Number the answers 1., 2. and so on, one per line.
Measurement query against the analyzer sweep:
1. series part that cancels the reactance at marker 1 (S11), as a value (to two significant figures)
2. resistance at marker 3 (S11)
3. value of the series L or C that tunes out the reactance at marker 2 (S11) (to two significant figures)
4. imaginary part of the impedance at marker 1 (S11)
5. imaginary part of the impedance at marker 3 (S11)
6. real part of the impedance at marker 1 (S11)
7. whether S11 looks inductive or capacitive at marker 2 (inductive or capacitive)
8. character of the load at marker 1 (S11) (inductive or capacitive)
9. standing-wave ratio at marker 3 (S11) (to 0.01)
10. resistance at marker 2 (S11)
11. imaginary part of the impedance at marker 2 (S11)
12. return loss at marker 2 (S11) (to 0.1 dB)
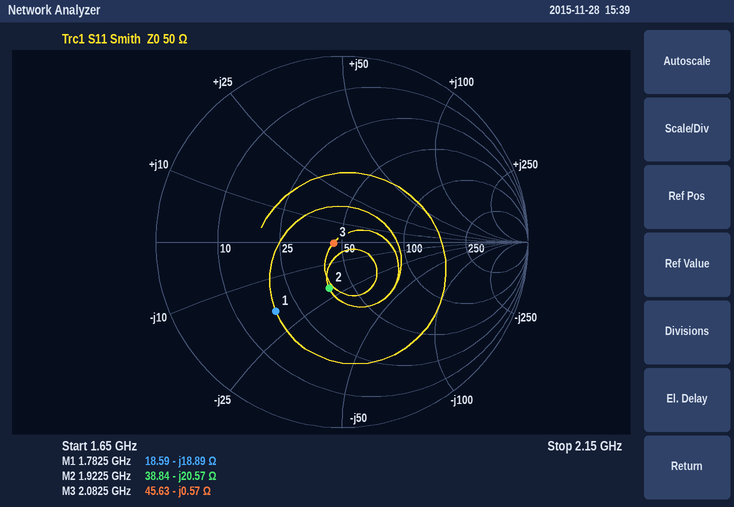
1. 1.7 nH
2. 45.63 Ω
3. 1.7 nH
4. -18.89 Ω
5. -0.57 Ω
6. 18.59 Ω
7. capacitive
8. capacitive
9. 1.10
10. 38.84 Ω
11. -20.57 Ω
12. 11.8 dB
